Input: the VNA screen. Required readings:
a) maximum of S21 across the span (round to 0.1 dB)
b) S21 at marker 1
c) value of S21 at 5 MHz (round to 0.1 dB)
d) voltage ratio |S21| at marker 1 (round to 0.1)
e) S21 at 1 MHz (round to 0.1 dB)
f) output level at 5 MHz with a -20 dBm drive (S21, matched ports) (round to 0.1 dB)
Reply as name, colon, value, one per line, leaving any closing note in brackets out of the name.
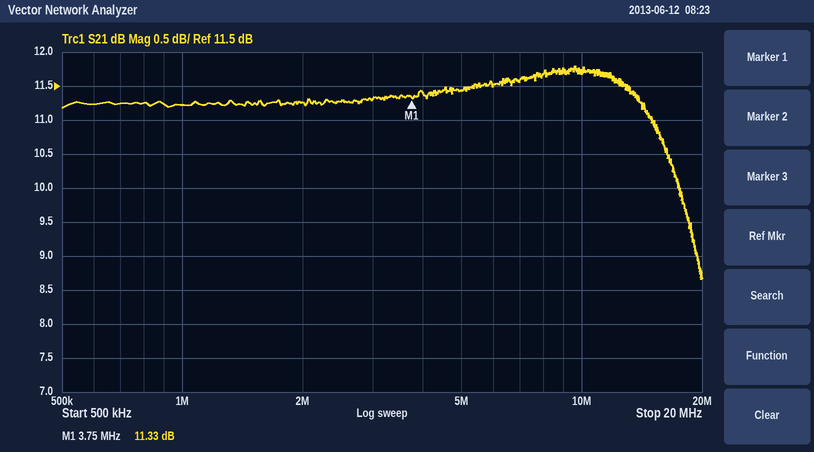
maximum of S21 across the span: 11.8 dB
S21 at marker 1: 11.33 dB
value of S21 at 5 MHz: 11.4 dB
voltage ratio |S21| at marker 1: 3.7
S21 at 1 MHz: 11.2 dB
output level at 5 MHz with a -20 dBm drive (S21, matched ports): -8.6 dBm
